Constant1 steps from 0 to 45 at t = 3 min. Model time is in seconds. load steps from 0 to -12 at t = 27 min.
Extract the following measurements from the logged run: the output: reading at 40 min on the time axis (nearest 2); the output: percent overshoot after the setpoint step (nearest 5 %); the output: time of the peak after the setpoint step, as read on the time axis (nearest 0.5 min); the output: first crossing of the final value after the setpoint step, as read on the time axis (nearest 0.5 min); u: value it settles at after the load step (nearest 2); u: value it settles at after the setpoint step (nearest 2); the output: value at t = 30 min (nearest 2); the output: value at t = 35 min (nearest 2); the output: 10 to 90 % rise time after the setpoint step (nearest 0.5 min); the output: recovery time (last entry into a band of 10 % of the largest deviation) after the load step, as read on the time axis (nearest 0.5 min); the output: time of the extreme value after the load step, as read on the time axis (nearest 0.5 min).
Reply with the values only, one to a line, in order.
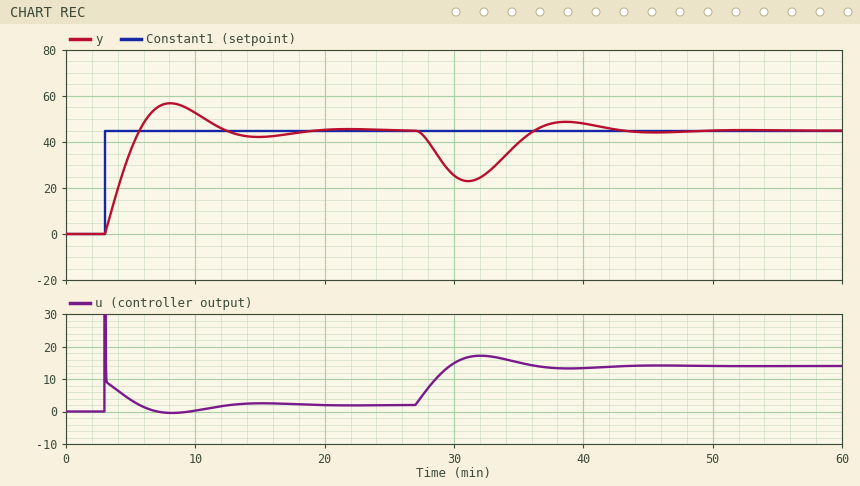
48
25 %
8.0 min
5.5 min
14
2
26
40
2.0 min
41.0 min
31.0 min
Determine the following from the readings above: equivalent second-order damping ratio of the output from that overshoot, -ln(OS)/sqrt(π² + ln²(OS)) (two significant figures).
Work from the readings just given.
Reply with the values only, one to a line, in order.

0.40
